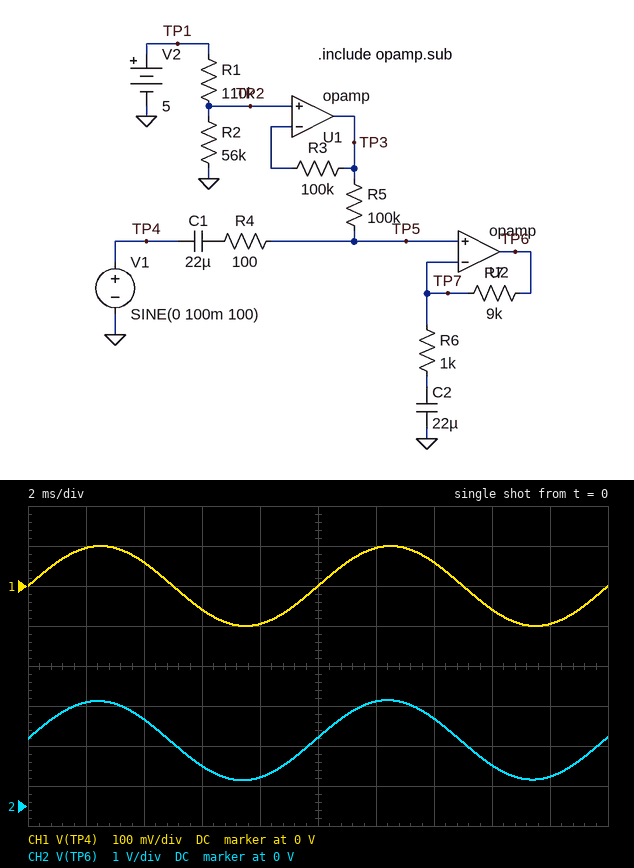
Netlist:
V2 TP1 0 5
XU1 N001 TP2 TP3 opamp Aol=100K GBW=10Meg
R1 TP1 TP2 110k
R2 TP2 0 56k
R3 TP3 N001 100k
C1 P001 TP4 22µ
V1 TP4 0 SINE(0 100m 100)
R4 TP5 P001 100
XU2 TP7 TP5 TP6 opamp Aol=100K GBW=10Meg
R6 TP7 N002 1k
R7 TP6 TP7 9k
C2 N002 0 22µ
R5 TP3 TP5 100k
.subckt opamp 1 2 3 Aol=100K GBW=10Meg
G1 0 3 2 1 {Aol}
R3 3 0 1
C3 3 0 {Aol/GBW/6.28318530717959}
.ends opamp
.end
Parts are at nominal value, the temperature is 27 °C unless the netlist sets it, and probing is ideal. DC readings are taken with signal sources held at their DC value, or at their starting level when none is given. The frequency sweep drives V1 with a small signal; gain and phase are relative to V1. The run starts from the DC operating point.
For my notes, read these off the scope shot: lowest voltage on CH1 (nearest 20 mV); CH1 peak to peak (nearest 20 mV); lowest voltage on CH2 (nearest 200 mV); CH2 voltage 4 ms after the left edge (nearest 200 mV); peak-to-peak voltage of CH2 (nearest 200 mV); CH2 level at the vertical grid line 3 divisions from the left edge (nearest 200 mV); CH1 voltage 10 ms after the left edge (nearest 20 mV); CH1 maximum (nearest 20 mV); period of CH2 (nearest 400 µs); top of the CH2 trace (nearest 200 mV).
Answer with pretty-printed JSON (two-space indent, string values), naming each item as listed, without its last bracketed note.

{
  "lowest voltage on CH1": "-100 mV",
  "CH1 peak to peak": "200 mV",
  "lowest voltage on CH2": "600 mV",
  "CH2 voltage 4 ms after the left edge": "2.2 V",
  "peak-to-peak voltage of CH2": "2.0 V",
  "CH2 level at the vertical grid line 3 divisions from the left edge": "1.0 V",
  "CH1 voltage 10 ms after the left edge": "0 V",
  "CH1 maximum": "100 mV",
  "period of CH2": "10.0 ms",
  "top of the CH2 trace": "2.6 V"
}
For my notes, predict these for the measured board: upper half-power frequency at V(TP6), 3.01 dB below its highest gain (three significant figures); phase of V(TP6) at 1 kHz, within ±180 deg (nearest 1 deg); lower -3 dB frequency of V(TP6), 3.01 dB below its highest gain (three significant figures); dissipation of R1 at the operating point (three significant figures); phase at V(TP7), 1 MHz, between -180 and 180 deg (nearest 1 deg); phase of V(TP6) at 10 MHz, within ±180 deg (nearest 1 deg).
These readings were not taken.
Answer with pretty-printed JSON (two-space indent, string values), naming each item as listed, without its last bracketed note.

{
  "upper half-power frequency at V(TP6), 3.01 dB below its highest gain": "1.00 MHz",
  "phase of V(TP6) at 1 kHz, within ±180 deg": "0 deg",
  "lower -3 dB frequency of V(TP6), 3.01 dB below its highest gain": "7.16 Hz",
  "dissipation of R1 at the operating point": "99.8 µW",
  "phase at V(TP7), 1 MHz, between -180 and 180 deg": "-45 deg",
  "phase of V(TP6) at 10 MHz, within ±180 deg": "-84 deg"
}
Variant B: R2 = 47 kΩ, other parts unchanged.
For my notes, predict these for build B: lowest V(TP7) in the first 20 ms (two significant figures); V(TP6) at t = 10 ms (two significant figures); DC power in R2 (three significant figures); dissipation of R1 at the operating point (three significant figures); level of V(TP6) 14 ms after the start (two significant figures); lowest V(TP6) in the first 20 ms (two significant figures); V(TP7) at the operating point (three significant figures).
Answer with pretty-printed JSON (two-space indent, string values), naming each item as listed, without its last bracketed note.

{
  "lowest V(TP7) in the first 20 ms": "1.4 V",
  "V(TP6) at t = 10 ms": "1.5 V",
  "DC power in R2": "47.7 µW",
  "dissipation of R1 at the operating point": "112 µW",
  "level of V(TP6) 14 ms after the start": "2.0 V",
  "lowest V(TP6) in the first 20 ms": "450 mV",
  "V(TP7) at the operating point": "1.50 V"
}
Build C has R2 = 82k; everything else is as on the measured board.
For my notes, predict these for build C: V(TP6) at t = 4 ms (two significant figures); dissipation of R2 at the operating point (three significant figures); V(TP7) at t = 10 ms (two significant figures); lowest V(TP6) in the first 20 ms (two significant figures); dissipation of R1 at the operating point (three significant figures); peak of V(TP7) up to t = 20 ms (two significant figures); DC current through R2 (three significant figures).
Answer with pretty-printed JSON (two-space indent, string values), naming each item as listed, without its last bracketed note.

{
  "V(TP6) at t = 4 ms": "2.6 V",
  "dissipation of R2 at the operating point": "55.6 µW",
  "V(TP7) at t = 10 ms": "2.1 V",
  "lowest V(TP6) in the first 20 ms": "1.1 V",
  "dissipation of R1 at the operating point": "74.6 µW",
  "peak of V(TP7) up to t = 20 ms": "2.2 V",
  "DC current through R2": "26.0 µA"
}
